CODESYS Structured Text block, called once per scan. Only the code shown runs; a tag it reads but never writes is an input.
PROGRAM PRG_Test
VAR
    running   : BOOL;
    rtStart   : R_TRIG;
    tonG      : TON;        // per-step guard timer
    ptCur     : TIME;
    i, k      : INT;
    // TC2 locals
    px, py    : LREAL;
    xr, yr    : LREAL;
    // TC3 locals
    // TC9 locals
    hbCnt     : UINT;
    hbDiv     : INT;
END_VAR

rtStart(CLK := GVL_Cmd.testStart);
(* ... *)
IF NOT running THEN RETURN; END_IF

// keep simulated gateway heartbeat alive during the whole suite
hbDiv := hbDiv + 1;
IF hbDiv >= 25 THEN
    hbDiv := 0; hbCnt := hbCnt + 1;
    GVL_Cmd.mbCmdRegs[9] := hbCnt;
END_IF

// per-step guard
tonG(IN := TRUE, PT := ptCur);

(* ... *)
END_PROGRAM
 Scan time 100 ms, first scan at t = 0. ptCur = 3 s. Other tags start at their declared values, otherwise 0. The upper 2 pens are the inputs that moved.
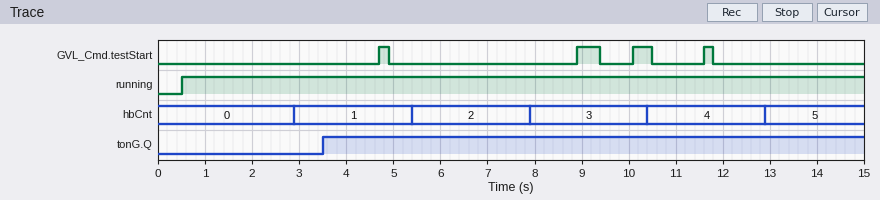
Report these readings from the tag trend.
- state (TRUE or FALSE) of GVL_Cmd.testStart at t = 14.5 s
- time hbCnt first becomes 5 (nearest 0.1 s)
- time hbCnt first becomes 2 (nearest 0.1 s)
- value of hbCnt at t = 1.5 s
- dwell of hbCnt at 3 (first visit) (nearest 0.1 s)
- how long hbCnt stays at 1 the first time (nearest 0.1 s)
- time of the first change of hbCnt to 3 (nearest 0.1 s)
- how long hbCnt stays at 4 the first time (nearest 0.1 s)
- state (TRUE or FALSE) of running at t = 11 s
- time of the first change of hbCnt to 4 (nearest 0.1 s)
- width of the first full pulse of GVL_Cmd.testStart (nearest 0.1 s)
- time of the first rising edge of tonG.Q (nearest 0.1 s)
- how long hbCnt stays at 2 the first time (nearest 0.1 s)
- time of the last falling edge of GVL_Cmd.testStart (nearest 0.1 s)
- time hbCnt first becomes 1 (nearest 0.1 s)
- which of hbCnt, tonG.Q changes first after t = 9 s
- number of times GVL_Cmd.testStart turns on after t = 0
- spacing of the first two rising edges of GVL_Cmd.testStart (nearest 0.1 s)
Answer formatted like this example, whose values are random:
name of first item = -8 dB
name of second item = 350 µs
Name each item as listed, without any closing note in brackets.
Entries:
state (TRUE or FALSE) of GVL_Cmd.testStart at t = 14.5 s = FALSE
time hbCnt first becomes 5 = 12.9 s
time hbCnt first becomes 2 = 5.4 s
value of hbCnt at t = 1.5 s = 0
dwell of hbCnt at 3 (first visit) = 2.5 s
how long hbCnt stays at 1 the first time = 2.5 s
time of the first change of hbCnt to 3 = 7.9 s
how long hbCnt stays at 4 the first time = 2.5 s
state (TRUE or FALSE) of running at t = 11 s = TRUE
time of the first change of hbCnt to 4 = 10.4 s
width of the first full pulse of GVL_Cmd.testStart = 0.2 s
time of the first rising edge of tonG.Q = 3.5 s
how long hbCnt stays at 2 the first time = 2.5 s
time of the last falling edge of GVL_Cmd.testStart = 11.8 s
time hbCnt first becomes 1 = 2.9 s
which of hbCnt, tonG.Q changes first after t = 9 s = hbCnt
number of times GVL_Cmd.testStart turns on after t = 0 = 4
spacing of the first two rising edges of GVL_Cmd.testStart = 4.2 s
